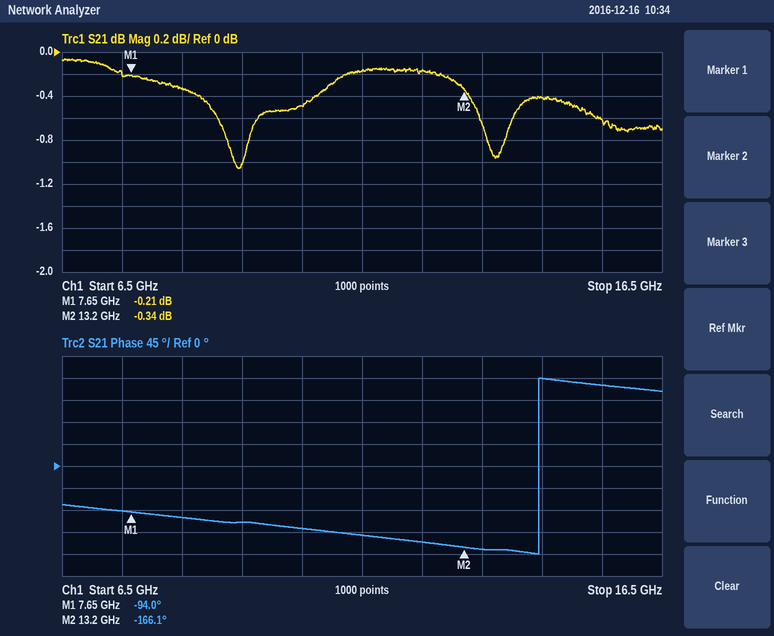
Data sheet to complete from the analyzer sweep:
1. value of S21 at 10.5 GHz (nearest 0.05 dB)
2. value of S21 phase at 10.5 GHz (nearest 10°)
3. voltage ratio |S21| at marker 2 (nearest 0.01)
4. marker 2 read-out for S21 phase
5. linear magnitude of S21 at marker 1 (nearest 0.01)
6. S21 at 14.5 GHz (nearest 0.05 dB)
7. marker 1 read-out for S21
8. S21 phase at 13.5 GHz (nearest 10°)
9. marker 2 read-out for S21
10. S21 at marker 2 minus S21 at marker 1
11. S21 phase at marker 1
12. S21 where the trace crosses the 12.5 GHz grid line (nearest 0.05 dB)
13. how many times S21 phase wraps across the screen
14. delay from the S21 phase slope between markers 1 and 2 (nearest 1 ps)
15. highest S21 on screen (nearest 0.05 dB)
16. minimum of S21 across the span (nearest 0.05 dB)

-0.50 dB
-130°
0.96
-166.1°
0.98
-0.40 dB
-0.21 dB
-170°
-0.34 dB
-0.13 dB
-94.0°
-0.15 dB
1
36 ps
-0.05 dB
-1.05 dB
